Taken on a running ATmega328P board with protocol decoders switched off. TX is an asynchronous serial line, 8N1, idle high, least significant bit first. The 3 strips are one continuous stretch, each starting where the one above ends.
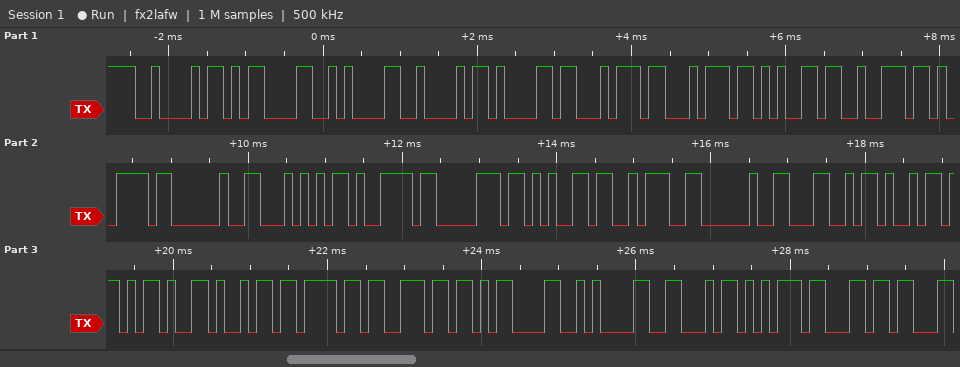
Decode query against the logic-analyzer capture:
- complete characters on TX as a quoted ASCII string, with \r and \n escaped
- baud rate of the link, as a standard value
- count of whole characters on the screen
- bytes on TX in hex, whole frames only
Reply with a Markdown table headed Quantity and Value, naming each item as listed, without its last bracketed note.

| Quantity | Value |
|---|---|
| complete characters on TX as a quoted ASCII string, with \r and \n escaped | "B\r\nBattery Type: Li-ion\r\nFul" |
| baud rate of the link, as a standard value | 9600 baud |
| count of whole characters on the screen | 28 |
| bytes on TX in hex, whole frames only | 42 0D 0A 42 61 74 74 65 72 79 20 54 79 70 65 3A 20 4C 69 2D 69 6F 6E 0D 0A 46 75 6C |
